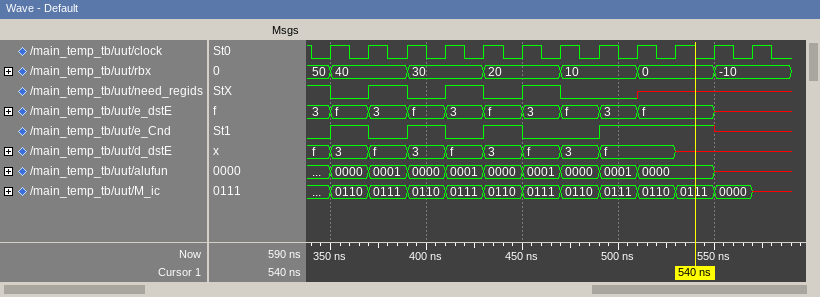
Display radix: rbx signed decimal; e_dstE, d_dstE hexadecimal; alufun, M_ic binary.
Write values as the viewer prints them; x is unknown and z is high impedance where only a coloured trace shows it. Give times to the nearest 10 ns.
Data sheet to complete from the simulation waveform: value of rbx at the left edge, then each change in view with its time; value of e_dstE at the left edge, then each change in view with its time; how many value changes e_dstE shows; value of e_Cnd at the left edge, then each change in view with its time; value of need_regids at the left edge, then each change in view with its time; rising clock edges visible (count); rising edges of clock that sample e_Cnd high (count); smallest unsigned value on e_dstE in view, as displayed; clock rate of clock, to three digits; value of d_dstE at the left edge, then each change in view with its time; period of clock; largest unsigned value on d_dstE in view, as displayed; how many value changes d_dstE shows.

50, 40 at 350 ns, 30 at 390 ns, 20 at 430 ns, 10 at 470 ns, 0 at 510 ns, -10 at 550 ns
3, f at 350 ns, 3 at 370 ns, f at 390 ns, 3 at 410 ns, f at 430 ns, 3 at 450 ns, f at 470 ns, 3 at 490 ns, f at 510 ns, x at 550 ns
10
0, 1 at 350 ns, 0 at 370 ns, 1 at 390 ns, 0 at 410 ns, 1 at 430 ns, 0 at 450 ns, 1 at 490 ns, x at 550 ns
1, 0 at 350 ns, 1 at 370 ns, 0 at 390 ns, 1 at 410 ns, 0 at 430 ns, 1 at 450 ns, 0 at 470 ns, x at 510 ns
12
6
3
50.0 MHz
f, 3 at 350 ns, f at 370 ns, 3 at 390 ns, f at 410 ns, 3 at 430 ns, f at 450 ns, 3 at 470 ns, f at 490 ns, x at 530 ns
20 ns
f
9
